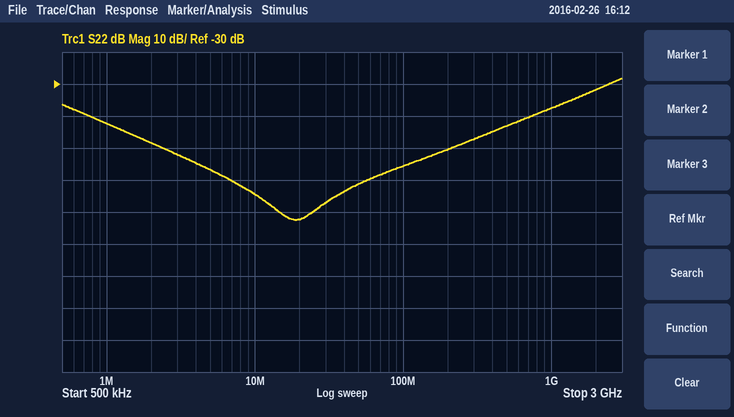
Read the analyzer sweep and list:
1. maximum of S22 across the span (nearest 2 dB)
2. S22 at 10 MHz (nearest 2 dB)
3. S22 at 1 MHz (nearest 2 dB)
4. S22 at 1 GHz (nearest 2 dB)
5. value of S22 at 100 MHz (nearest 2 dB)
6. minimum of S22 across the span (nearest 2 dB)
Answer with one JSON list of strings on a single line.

["-28 dB", "-64 dB", "-42 dB", "-38 dB", "-56 dB", "-72 dB"]
